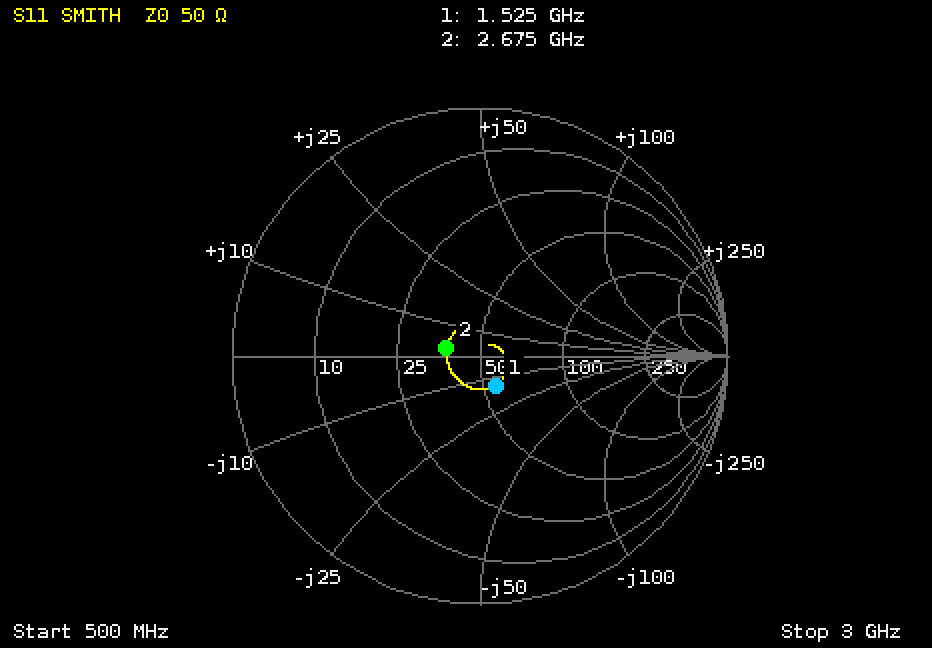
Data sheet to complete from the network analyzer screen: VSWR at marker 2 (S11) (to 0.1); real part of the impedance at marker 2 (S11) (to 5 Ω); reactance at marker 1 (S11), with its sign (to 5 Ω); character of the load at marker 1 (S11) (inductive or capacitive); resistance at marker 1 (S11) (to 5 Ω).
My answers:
1.3
40 Ω
-15 Ω
capacitive
55 Ω
